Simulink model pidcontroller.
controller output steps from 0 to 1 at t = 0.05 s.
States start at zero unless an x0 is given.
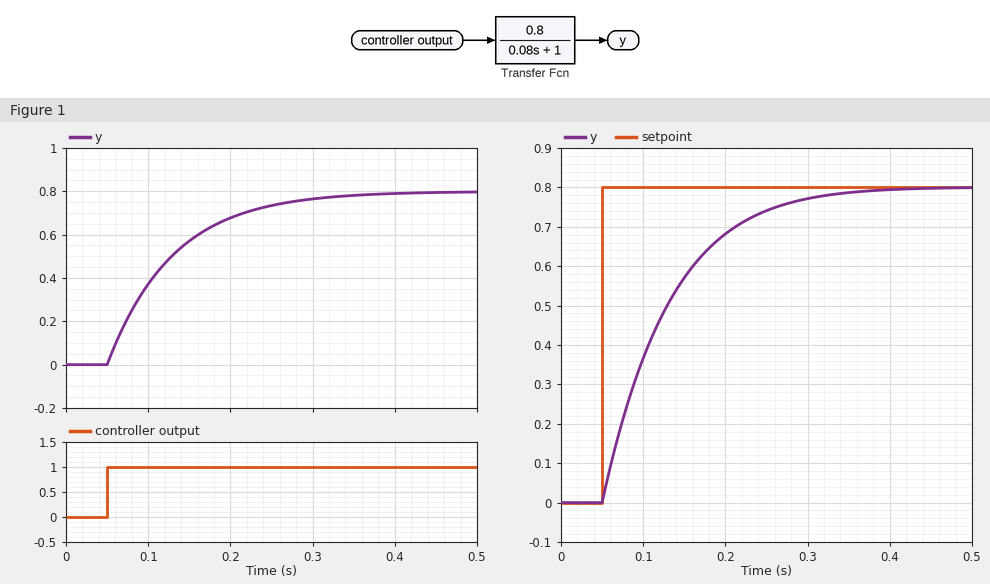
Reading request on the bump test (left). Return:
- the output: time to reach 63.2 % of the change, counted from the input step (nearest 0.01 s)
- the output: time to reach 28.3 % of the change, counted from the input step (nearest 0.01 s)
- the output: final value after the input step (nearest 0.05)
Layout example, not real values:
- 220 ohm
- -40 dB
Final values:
- 0.08 s
- 0.03 s
- 0.80
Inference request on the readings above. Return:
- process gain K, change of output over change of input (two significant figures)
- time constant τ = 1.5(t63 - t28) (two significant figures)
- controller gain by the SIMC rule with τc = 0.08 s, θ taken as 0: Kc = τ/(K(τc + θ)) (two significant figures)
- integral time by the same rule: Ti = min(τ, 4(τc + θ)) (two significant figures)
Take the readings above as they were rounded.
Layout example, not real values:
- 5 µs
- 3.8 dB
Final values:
- 0.80
- 0.075 s
- 1.2
- 0.075 s
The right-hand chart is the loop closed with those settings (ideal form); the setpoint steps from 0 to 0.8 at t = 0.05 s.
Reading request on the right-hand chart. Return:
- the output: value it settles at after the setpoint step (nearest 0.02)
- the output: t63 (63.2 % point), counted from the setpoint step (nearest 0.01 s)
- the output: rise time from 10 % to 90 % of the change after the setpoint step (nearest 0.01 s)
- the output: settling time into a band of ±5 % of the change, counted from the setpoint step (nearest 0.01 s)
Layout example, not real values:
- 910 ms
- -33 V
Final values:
- 0.80
- 0.08 s
- 0.17 s
- 0.23 s
